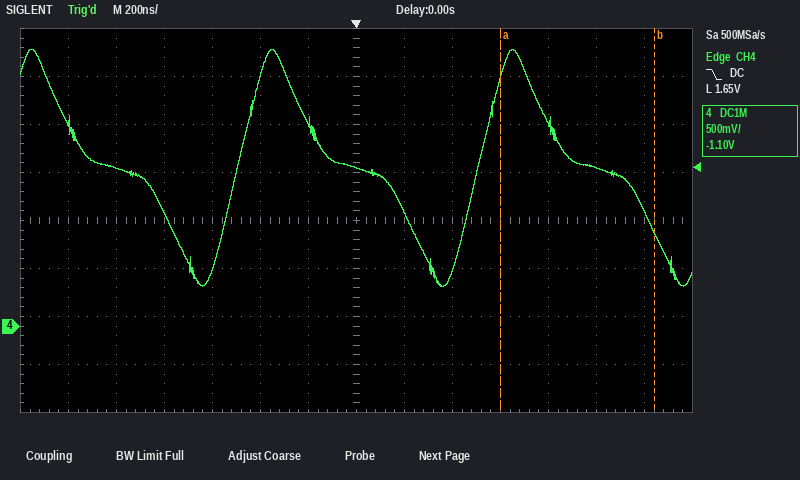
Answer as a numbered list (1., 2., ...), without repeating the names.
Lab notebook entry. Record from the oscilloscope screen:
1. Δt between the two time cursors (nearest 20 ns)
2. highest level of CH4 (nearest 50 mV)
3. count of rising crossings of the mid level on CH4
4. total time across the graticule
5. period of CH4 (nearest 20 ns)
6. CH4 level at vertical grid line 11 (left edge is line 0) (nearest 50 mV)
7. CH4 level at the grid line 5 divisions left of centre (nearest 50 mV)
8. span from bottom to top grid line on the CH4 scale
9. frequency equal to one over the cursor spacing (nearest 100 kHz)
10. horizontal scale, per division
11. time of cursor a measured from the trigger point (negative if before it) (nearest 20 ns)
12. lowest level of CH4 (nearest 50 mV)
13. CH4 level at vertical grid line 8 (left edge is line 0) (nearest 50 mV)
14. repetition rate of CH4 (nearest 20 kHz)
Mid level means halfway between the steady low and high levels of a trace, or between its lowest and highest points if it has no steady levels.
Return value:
1. 640 ns
2. 2.90 V
3. 2
4. 2.8 µs
5. 1.00 µs
6. 2.10 V
7. 1.65 V
8. 4 V
9. 1.6 MHz
10. 200 ns
11. +600 ns
12. 400 mV
13. 1.20 V
14. 1.00 MHz
